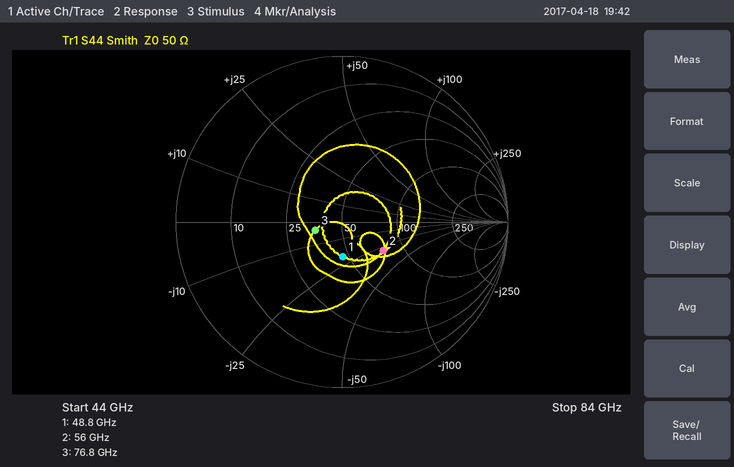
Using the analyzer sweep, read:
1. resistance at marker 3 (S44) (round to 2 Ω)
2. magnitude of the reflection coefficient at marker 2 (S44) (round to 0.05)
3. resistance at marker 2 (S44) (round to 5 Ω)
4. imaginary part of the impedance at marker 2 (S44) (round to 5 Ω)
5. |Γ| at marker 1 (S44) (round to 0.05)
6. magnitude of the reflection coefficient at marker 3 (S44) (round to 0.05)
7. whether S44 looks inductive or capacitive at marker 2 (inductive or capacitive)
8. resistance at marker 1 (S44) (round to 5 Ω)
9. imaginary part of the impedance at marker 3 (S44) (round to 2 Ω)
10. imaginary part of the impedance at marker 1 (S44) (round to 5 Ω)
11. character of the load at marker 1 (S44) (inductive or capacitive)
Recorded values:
36 Ω
0.30
75 Ω
-30 Ω
0.20
0.15
capacitive
45 Ω
-4 Ω
-20 Ω
capacitive
